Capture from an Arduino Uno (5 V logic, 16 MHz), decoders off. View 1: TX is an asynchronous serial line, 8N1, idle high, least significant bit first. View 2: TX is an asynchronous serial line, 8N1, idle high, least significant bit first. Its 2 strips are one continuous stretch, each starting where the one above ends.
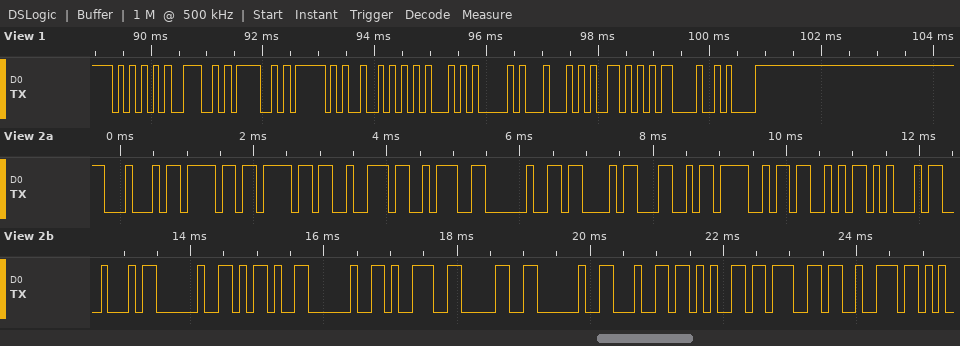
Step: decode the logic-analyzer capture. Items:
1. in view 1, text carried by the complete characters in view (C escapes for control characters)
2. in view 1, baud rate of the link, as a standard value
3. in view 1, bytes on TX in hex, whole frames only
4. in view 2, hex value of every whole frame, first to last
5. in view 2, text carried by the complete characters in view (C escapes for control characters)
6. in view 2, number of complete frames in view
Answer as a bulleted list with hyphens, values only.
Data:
- "UNO_READY\r\n"
- 9600 baud
- 55 4E 4F 5F 52 45 41 44 59 0D 0A
- 44 6F 6F 72 3A 20 43 4C 4F 53 45 44 20 2D 20 39 30 20 64 65 67 72
- "Door: CLOSED - 90 degr"
- 22
